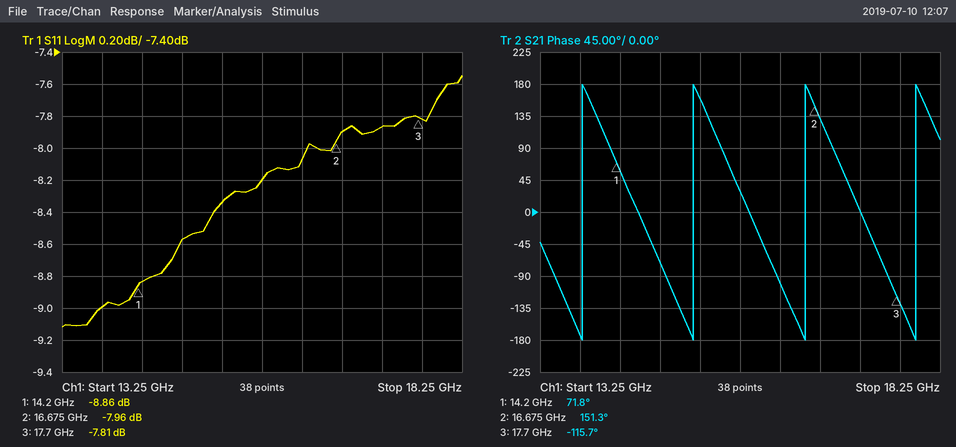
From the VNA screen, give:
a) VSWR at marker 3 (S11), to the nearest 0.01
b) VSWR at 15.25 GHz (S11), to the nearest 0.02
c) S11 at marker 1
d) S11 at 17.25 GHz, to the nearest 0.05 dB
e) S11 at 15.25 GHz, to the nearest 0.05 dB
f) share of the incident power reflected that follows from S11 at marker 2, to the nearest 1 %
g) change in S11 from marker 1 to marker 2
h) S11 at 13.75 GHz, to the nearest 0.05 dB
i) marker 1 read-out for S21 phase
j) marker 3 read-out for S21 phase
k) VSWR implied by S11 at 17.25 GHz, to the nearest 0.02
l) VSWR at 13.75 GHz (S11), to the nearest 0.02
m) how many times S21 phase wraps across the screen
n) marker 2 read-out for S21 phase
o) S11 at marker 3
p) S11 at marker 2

2.37
2.24
-8.86 dB
-7.85 dB
-8.35 dB
16 %
0.90 dB
-9.00 dB
71.8°
-115.7°
2.36
2.10
4
151.3°
-7.81 dB
-7.96 dB
